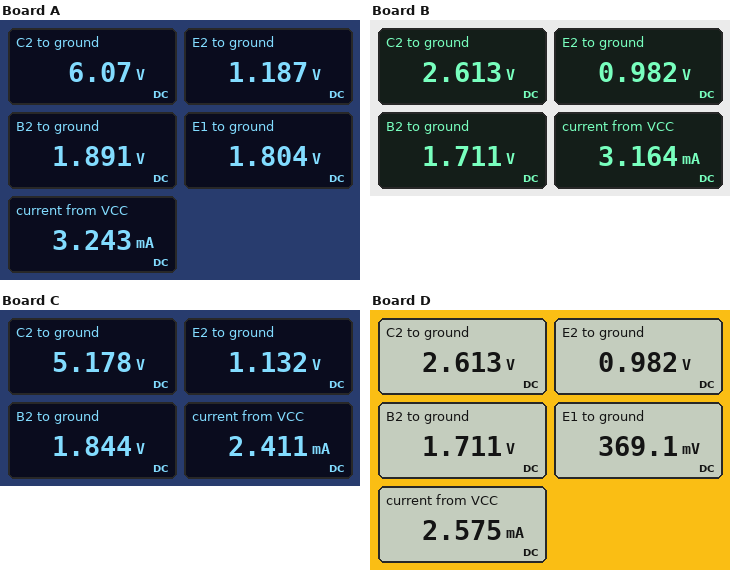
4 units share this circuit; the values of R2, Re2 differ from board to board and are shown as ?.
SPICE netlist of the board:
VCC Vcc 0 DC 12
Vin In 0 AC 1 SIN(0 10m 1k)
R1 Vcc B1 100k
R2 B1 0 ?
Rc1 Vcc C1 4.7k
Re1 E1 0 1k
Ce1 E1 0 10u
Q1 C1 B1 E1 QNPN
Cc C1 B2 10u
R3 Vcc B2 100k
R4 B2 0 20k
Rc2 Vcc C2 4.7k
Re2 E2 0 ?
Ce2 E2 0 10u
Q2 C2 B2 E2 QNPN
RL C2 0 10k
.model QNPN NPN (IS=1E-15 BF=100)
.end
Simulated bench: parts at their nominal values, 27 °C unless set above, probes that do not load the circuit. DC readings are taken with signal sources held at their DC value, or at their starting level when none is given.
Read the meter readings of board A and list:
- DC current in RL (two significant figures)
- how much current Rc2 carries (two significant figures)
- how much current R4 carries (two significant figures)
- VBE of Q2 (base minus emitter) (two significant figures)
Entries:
610 µA
1.3 mA
95 µA
700 mV
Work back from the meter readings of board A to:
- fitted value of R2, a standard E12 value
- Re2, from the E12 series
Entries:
33 kΩ
1.8 kΩ
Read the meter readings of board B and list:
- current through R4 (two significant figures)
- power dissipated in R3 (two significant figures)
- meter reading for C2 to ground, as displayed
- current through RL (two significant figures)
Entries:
86 µA
1.1 mW
2.613 V
260 µA
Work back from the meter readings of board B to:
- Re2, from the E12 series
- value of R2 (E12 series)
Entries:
560 Ω
18 kΩ
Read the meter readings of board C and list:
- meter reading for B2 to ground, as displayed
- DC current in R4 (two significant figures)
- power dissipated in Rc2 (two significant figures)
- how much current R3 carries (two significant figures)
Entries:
1.844 V
92 µA
9.9 mW
100 µA
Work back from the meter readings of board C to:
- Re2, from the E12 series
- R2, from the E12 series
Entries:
1.2 kΩ
15 kΩ
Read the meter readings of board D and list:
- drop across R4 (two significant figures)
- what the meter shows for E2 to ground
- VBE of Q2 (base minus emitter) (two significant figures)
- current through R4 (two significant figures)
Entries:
1.7 V
0.982 V
730 mV
86 µA
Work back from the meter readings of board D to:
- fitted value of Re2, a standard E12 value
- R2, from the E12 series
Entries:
560 Ω
10 kΩ
